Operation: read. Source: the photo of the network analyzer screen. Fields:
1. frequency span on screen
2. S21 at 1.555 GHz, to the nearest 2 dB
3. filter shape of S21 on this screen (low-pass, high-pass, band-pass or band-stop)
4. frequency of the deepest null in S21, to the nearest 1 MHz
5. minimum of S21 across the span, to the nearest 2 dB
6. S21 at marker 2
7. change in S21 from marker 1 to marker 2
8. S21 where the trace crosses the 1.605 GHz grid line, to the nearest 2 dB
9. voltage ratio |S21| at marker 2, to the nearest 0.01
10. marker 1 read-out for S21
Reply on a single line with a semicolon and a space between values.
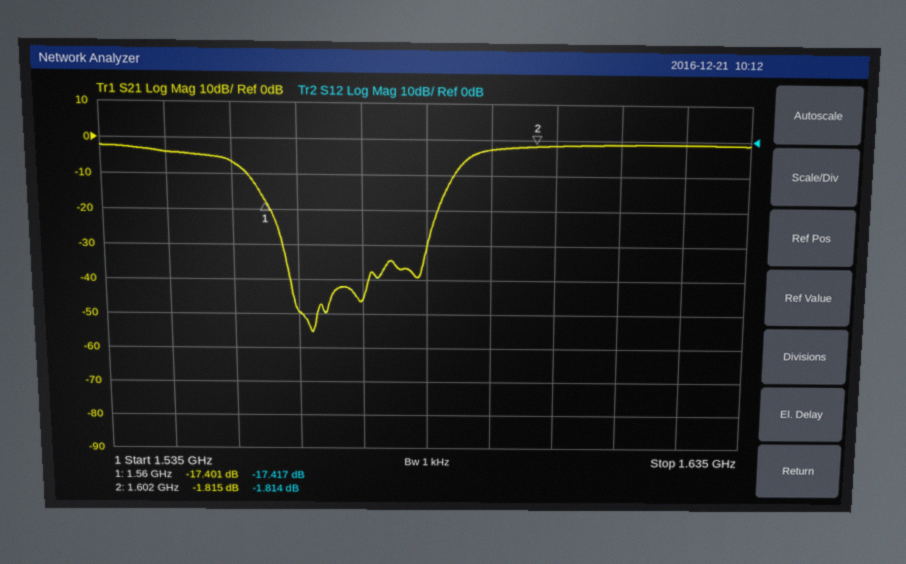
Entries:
100 MHz; -6 dB; band-stop; 1.567 GHz; -56 dB; -1.815 dB; 15.586 dB; -2 dB; 0.81; -17.401 dB
